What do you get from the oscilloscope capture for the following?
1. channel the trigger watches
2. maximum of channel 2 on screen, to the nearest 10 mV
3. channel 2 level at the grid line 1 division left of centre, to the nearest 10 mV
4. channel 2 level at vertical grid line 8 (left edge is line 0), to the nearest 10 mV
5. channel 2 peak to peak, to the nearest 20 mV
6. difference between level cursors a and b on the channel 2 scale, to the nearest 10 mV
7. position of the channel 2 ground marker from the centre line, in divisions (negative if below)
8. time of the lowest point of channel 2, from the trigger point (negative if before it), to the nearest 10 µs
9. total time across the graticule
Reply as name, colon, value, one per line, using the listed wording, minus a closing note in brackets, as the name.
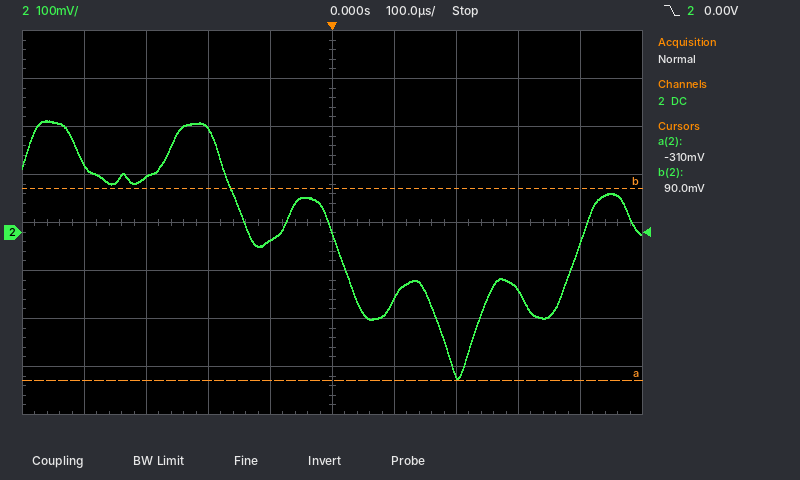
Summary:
channel the trigger watches: channel 2
maximum of channel 2 on screen, to the nearest 10 mV: 230 mV
channel 2 level at the grid line 1 division left of centre, to the nearest 10 mV: -20 mV
channel 2 level at vertical grid line 8 (left edge is line 0), to the nearest 10 mV: -120 mV
channel 2 peak to peak, to the nearest 20 mV: 540 mV
difference between level cursors a and b on the channel 2 scale, to the nearest 10 mV: 400 mV
position of the channel 2 ground marker from the centre line, in divisions: -0.2 div
time of the lowest point of channel 2, from the trigger point (negative if before it), to the nearest 10 µs: +200 µs
total time across the graticule: 1 ms
